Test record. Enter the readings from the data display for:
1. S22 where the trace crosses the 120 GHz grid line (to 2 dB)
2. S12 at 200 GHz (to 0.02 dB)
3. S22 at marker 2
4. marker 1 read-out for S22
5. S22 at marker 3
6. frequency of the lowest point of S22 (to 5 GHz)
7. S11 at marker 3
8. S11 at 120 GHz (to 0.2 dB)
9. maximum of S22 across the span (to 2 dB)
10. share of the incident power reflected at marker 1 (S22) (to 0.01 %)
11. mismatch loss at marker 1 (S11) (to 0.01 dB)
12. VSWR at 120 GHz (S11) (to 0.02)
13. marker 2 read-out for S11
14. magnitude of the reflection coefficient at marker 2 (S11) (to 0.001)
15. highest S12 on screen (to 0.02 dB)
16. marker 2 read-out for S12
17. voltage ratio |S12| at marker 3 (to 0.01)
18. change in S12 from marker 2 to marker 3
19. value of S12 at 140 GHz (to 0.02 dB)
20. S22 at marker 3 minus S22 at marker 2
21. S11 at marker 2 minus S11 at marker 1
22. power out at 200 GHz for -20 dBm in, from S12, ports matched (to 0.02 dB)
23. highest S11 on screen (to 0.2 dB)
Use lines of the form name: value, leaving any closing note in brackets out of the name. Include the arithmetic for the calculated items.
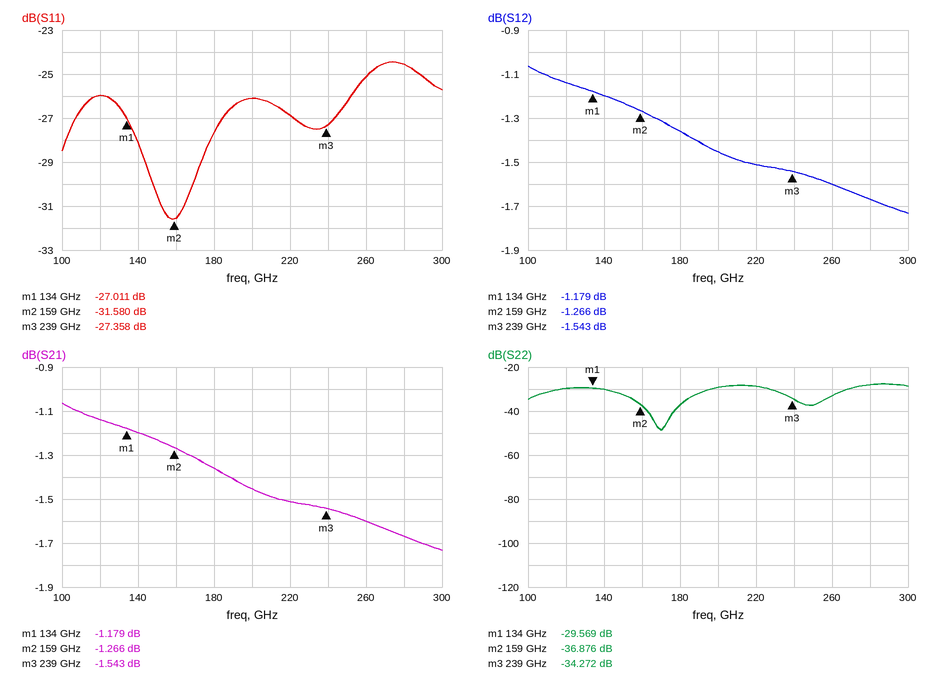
S22 where the trace crosses the 120 GHz grid line: -30 dB
S12 at 200 GHz: -1.46 dB
S22 at marker 2: -36.876 dB
marker 1 read-out for S22: -29.569 dB
S22 at marker 3: -34.272 dB
frequency of the lowest point of S22: 170 GHz
S11 at marker 3: -27.358 dB
S11 at 120 GHz: -26.0 dB
maximum of S22 across the span: -28 dB
share of the incident power reflected at marker 1 (S22): 10^(-29.569/10) ≈ 0.11 %
mismatch loss at marker 1 (S11): −10 log10(1 − 10^(-27.011/10)) ≈ 0.01 dB
VSWR at 120 GHz (S11): |Γ| = 10^(-26/20) = 0.0501; VSWR = (1 + 0.0501)/(1 − 0.0501) ≈ 1.11, so 1.10 to the nearest 0.02
marker 2 read-out for S11: -31.580 dB
magnitude of the reflection coefficient at marker 2 (S11): 10^(-31.58/20) ≈ 0.026
highest S12 on screen: -1.06 dB
marker 2 read-out for S12: -1.266 dB
voltage ratio |S12| at marker 3: 10^(-1.543/20) ≈ 0.84
change in S12 from marker 2 to marker 3: -1.543 − (-1.266) = -0.277 dB
value of S12 at 140 GHz: -1.20 dB
S22 at marker 3 minus S22 at marker 2: -34.272 − (-36.876) = 2.604 dB
S11 at marker 2 minus S11 at marker 1: -31.58 − (-27.011) = -4.569 dB
power out at 200 GHz for -20 dBm in, from S12, ports matched: -20 dBm + (-1.46 dB) = -21.46 dBm
highest S11 on screen: -24.4 dB
